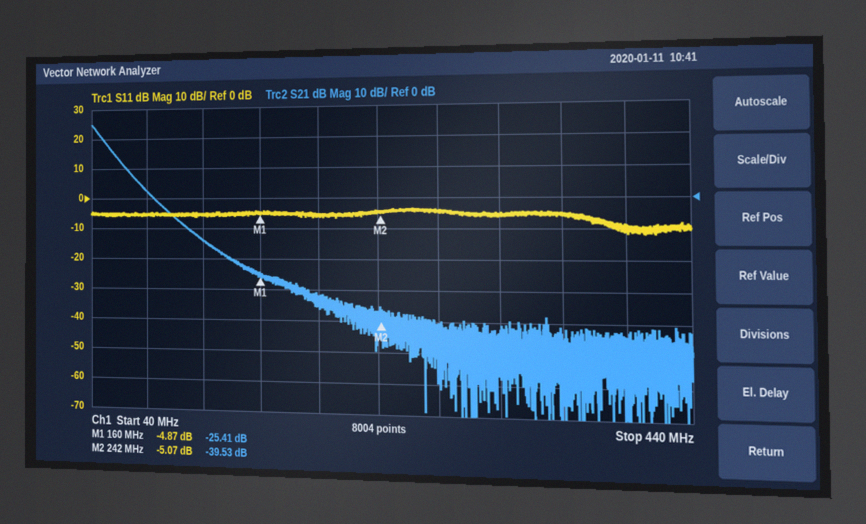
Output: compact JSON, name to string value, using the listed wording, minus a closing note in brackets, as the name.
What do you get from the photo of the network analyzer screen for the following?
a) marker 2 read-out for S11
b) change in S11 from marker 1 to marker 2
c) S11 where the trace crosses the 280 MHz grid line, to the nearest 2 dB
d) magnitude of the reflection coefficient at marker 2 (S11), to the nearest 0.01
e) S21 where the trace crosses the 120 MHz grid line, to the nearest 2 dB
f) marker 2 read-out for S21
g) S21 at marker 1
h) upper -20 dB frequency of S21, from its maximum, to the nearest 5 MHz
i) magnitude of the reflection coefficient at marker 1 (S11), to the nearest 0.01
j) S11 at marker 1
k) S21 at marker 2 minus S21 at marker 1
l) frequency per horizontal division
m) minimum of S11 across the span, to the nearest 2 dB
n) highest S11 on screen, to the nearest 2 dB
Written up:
{"marker 2 read-out for S11": "-5.07 dB", "change in S11 from marker 1 to marker 2": "-0.20 dB", "S11 where the trace crosses the 280 MHz grid line, to the nearest 2 dB": "-4 dB", "magnitude of the reflection coefficient at marker 2 (S11), to the nearest 0.01": "0.56", "S21 where the trace crosses the 120 MHz grid line, to the nearest 2 dB": "-14 dB", "marker 2 read-out for S21": "-39.53 dB", "S21 at marker 1": "-25.41 dB", "upper -20 dB frequency of S21, from its maximum, to the nearest 5 MHz": "75 MHz", "magnitude of the reflection coefficient at marker 1 (S11), to the nearest 0.01": "0.57", "S11 at marker 1": "-4.87 dB", "S21 at marker 2 minus S21 at marker 1": "-14.12 dB", "frequency per horizontal division": "40 MHz", "minimum of S11 across the span, to the nearest 2 dB": "-12 dB", "highest S11 on screen, to the nearest 2 dB": "-4 dB"}
